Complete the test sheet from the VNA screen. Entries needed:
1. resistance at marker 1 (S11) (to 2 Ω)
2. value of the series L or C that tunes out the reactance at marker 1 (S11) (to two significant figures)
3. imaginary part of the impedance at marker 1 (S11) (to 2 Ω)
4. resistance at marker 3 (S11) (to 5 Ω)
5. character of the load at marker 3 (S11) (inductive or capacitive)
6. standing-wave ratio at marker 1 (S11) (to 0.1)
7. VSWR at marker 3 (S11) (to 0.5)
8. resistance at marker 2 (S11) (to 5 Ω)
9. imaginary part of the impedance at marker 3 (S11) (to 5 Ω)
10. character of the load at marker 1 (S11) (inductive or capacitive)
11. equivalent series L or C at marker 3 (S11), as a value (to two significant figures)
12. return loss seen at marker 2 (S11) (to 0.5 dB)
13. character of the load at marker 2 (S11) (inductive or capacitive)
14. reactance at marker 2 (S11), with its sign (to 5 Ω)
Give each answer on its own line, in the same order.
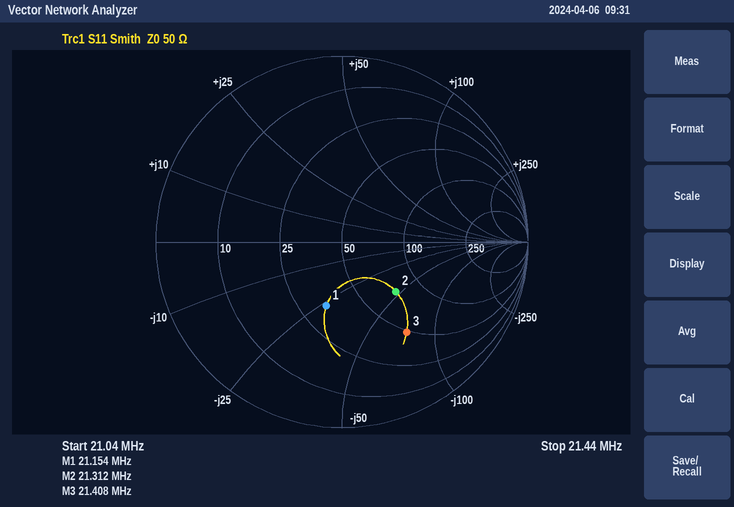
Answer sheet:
34 Ω
200 nH
-26 Ω
50 Ω
capacitive
2.1
4.0
75 Ω
-75 Ω
capacitive
100 pF
8.0 dB
capacitive
-45 Ω
